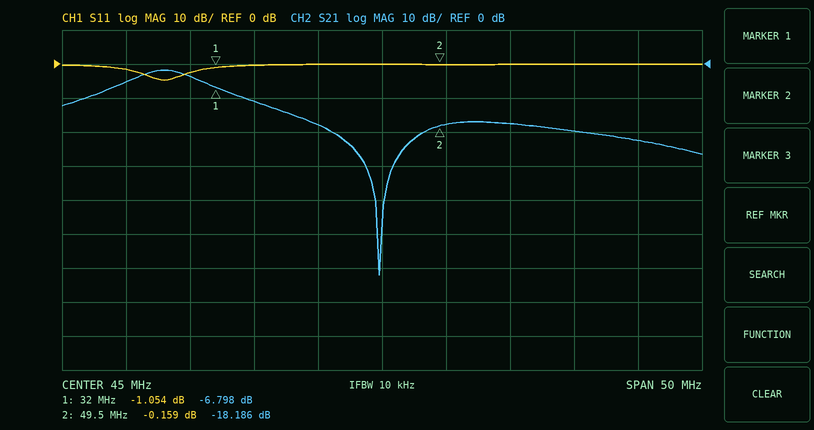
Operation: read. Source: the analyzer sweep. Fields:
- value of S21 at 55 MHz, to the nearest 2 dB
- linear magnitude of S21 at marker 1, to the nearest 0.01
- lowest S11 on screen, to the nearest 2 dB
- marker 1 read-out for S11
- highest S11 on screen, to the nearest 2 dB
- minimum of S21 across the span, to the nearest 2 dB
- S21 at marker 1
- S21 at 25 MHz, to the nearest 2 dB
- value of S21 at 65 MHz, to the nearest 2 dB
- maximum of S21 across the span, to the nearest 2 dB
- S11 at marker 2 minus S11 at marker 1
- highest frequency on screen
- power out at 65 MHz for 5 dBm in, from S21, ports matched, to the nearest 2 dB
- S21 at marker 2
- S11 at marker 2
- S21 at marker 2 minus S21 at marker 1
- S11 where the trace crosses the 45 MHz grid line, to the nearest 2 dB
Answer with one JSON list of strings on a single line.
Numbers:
["-18 dB", "0.46", "-4 dB", "-1.054 dB", "0 dB", "-62 dB", "-6.798 dB", "-6 dB", "-22 dB", "-2 dB", "0.895 dB", "70 MHz", "-18 dBm", "-18.186 dB", "-0.159 dB", "-11.388 dB", "0 dB"]
